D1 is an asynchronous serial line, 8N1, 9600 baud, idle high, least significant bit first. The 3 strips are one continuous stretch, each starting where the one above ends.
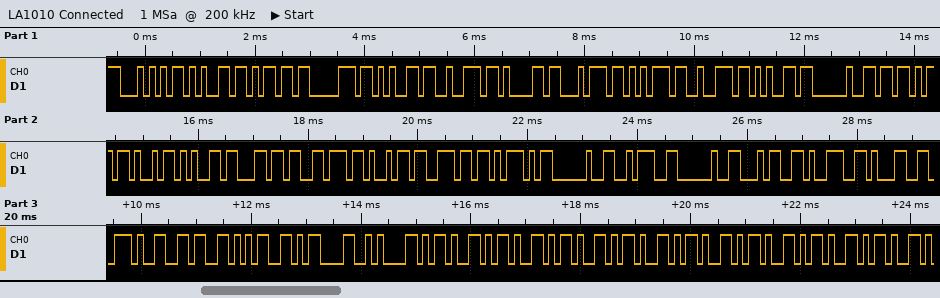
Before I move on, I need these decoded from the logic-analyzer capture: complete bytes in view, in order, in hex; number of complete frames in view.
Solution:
54 65 6D 70 65 72 61 74 75 72 65 20 5B 4B 65 6C 76 69 6E 5D 20 3A 20 34 39 31 2E 36 35 0D 0A 2D 2D 2D 2D 2D 2D 2D 2D
39
